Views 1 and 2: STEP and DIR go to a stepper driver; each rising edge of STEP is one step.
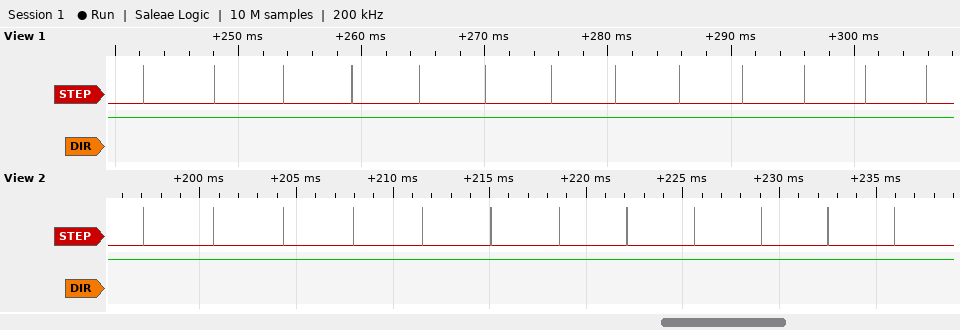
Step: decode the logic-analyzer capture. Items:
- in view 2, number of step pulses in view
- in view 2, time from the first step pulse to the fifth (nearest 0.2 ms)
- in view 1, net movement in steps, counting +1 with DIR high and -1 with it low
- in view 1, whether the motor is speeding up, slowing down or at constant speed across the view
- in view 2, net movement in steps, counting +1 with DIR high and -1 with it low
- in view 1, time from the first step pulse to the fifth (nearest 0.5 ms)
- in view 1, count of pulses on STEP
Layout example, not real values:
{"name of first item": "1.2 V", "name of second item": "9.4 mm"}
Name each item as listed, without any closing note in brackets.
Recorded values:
{"in view 2, number of step pulses in view": "12", "in view 2, time from the first step pulse to the fifth": "14.4 ms", "in view 1, net movement in steps, counting +1 with DIR high and -1 with it low": "+13", "in view 1, whether the motor is speeding up, slowing down or at constant speed across the view": "speeding up", "in view 2, net movement in steps, counting +1 with DIR high and -1 with it low": "+12", "in view 1, time from the first step pulse to the fifth": "22.5 ms", "in view 1, count of pulses on STEP": "13"}
